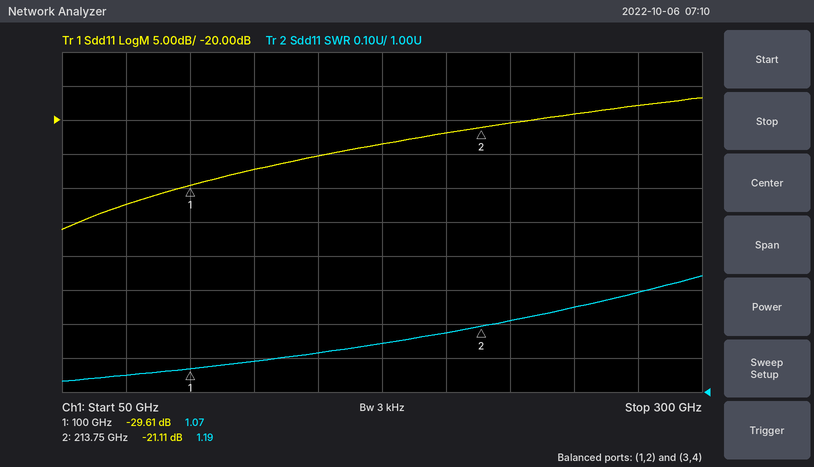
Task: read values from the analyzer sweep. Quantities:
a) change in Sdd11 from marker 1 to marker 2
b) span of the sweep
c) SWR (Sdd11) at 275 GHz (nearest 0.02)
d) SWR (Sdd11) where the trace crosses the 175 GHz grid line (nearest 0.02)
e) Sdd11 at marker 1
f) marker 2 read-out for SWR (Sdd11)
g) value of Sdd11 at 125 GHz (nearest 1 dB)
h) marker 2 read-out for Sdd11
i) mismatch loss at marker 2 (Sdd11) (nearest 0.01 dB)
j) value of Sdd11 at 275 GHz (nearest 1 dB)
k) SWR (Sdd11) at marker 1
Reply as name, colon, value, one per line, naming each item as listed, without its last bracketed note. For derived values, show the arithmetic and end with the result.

change in Sdd11 from marker 1 to marker 2: -21.11 − (-29.61) = 8.50 dB
span of the sweep: 250 GHz
SWR (Sdd11) at 275 GHz: 1.30
SWR (Sdd11) where the trace crosses the 175 GHz grid line: 1.14
Sdd11 at marker 1: -29.61 dB
marker 2 read-out for SWR: 1.19
value of Sdd11 at 125 GHz: -27 dB
marker 2 read-out for Sdd11: -21.11 dB
mismatch loss at marker 2 (Sdd11): −10 log10(1 − 10^(-21.11/10)) ≈ 0.03 dB
value of Sdd11 at 275 GHz: -18 dB
SWR (Sdd11) at marker 1: 1.07
